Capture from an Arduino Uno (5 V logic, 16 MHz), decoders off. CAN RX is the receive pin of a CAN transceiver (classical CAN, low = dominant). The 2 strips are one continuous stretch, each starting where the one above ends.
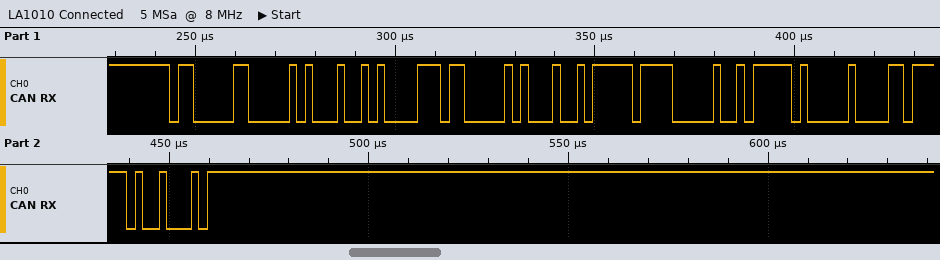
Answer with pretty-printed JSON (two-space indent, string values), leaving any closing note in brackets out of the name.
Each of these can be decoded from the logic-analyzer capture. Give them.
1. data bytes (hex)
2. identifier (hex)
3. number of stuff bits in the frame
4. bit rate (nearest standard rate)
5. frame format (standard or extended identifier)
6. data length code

{
  "data bytes": "94 3B 02 25 FF 01 7E 00",
  "identifier": "0x608",
  "number of stuff bits in the frame": "8",
  "bit rate": "500 kbit/s",
  "frame format": "standard",
  "data length code": "8"
}
